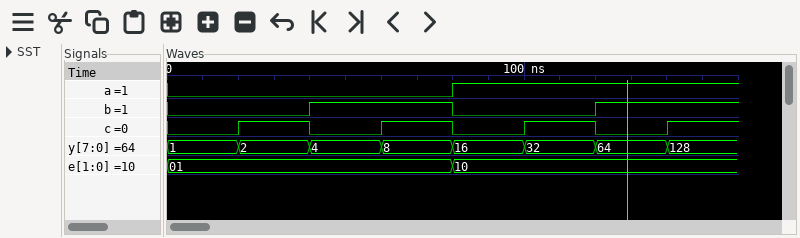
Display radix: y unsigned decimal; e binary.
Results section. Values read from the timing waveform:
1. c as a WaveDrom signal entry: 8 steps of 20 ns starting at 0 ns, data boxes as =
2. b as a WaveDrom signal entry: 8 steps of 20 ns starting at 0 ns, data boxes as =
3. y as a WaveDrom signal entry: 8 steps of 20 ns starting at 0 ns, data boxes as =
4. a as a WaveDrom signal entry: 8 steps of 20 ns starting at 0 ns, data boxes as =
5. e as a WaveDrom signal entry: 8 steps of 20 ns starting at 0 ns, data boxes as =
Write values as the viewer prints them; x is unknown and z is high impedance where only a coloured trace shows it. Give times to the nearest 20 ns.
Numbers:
{name: 'c', wave: '01010101'}
{name: 'b', wave: '0.1.0.1.'}
{name: 'y', wave: '========', data: '1 2 4 8 16 32 64 128'}
{name: 'a', wave: '0...1...'}
{name: 'e', wave: '=...=...', data: '01 10'}
